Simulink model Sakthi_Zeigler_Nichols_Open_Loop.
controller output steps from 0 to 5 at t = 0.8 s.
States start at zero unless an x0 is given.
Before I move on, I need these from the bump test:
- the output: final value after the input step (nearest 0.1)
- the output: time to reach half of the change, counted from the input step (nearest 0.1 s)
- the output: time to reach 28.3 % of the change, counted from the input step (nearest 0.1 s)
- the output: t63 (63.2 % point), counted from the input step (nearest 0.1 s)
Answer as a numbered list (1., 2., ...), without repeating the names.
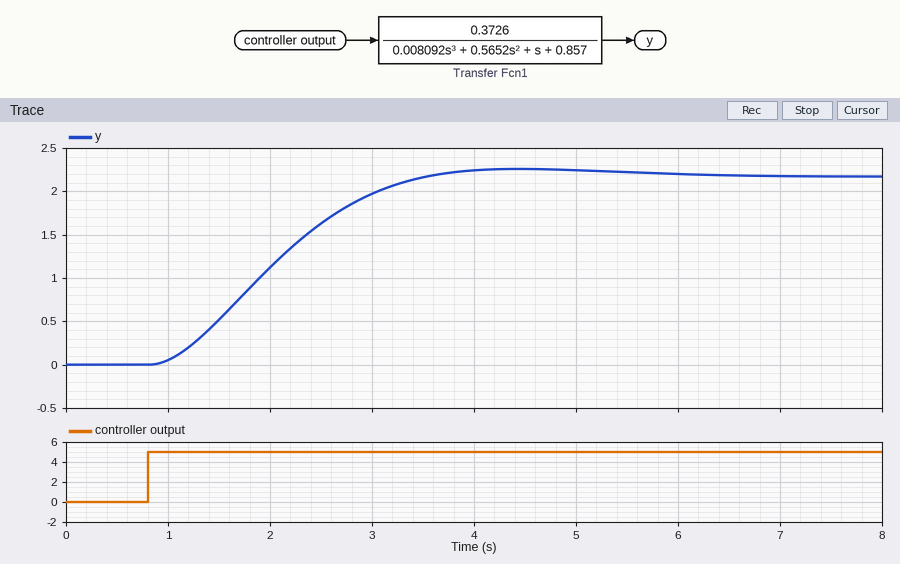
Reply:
1. 2.2
2. 1.2 s
3. 0.8 s
4. 1.4 s
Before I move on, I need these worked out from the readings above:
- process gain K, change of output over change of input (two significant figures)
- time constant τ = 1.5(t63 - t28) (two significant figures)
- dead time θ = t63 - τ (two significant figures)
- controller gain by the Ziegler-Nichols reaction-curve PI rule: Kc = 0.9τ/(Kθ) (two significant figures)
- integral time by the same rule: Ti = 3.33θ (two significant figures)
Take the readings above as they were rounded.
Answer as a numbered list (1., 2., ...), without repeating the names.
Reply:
1. 0.44
2. 0.90 s
3. 0.50 s
4. 3.7
5. 1.7 s
